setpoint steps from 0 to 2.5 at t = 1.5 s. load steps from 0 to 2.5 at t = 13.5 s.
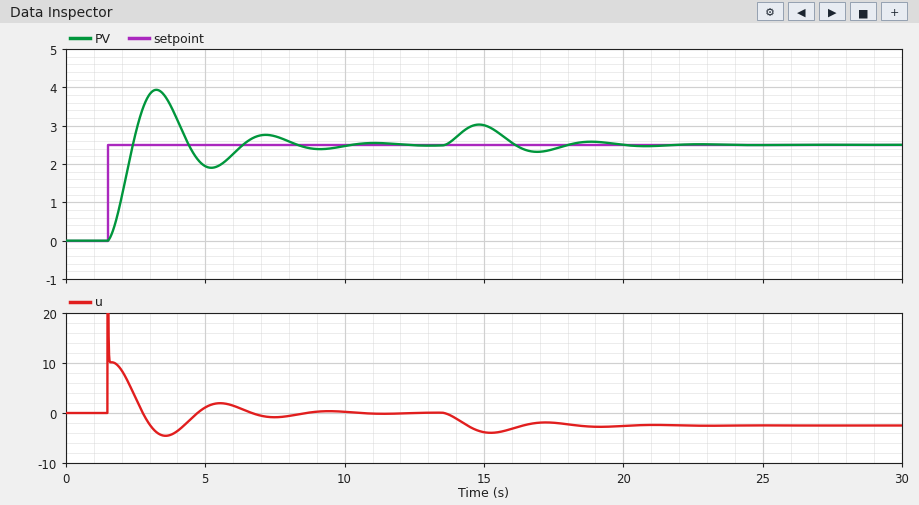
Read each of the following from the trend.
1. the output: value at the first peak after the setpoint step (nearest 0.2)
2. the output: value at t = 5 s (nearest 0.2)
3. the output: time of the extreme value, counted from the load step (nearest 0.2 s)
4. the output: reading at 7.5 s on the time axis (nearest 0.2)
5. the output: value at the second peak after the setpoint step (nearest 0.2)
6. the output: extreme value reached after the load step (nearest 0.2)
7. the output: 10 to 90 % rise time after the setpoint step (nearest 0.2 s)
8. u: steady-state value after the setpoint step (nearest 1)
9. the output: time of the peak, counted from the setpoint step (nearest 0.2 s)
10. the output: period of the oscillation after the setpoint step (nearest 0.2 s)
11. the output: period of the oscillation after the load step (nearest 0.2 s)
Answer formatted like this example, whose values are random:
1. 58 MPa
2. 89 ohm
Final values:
1. 4.0
2. 2.0
3. 1.4 s
4. 2.8
5. 2.8
6. 3.0
7. 0.6 s
8. 0
9. 1.8 s
10. 4.0 s
11. 4.0 s
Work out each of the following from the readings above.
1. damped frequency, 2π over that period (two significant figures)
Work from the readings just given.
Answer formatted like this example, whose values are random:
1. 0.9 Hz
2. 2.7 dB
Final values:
1. 1.6 rad/s
